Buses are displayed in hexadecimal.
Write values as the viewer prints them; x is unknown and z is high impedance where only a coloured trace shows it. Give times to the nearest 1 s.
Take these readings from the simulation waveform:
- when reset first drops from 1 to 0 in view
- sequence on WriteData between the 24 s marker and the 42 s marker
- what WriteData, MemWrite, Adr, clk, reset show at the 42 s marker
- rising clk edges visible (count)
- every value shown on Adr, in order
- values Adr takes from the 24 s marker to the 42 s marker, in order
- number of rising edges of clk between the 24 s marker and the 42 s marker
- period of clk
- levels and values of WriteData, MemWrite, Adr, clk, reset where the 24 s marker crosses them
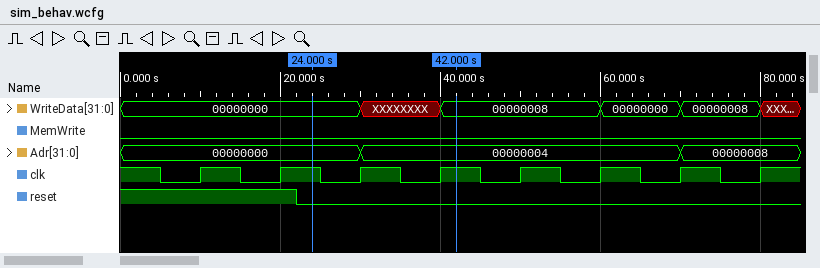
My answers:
22 s
00000000, XXXXXXXX, 00000008
WriteData=00000008, MemWrite=0, Adr=00000004, clk=1, reset=0
8
00000000, 00000004, 00000008
00000000, 00000004
2
10 s
WriteData=00000000, MemWrite=0, Adr=00000000, clk=1, reset=0
